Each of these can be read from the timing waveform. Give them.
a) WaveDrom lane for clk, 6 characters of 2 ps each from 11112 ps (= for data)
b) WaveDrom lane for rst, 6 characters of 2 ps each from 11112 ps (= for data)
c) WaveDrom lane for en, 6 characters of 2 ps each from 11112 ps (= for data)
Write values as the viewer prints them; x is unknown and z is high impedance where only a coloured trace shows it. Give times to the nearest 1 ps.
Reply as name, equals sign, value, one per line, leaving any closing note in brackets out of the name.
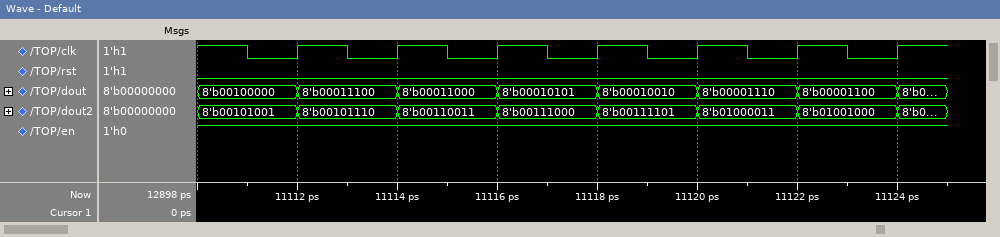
WaveDrom lane for clk, 6 characters of 2 ps each from 11112 ps = {name: 'clk', wave: 'p.....'}
WaveDrom lane for rst, 6 characters of 2 ps each from 11112 ps = {name: 'rst', wave: '0.....'}
WaveDrom lane for en, 6 characters of 2 ps each from 11112 ps = {name: 'en', wave: '1.....'}
